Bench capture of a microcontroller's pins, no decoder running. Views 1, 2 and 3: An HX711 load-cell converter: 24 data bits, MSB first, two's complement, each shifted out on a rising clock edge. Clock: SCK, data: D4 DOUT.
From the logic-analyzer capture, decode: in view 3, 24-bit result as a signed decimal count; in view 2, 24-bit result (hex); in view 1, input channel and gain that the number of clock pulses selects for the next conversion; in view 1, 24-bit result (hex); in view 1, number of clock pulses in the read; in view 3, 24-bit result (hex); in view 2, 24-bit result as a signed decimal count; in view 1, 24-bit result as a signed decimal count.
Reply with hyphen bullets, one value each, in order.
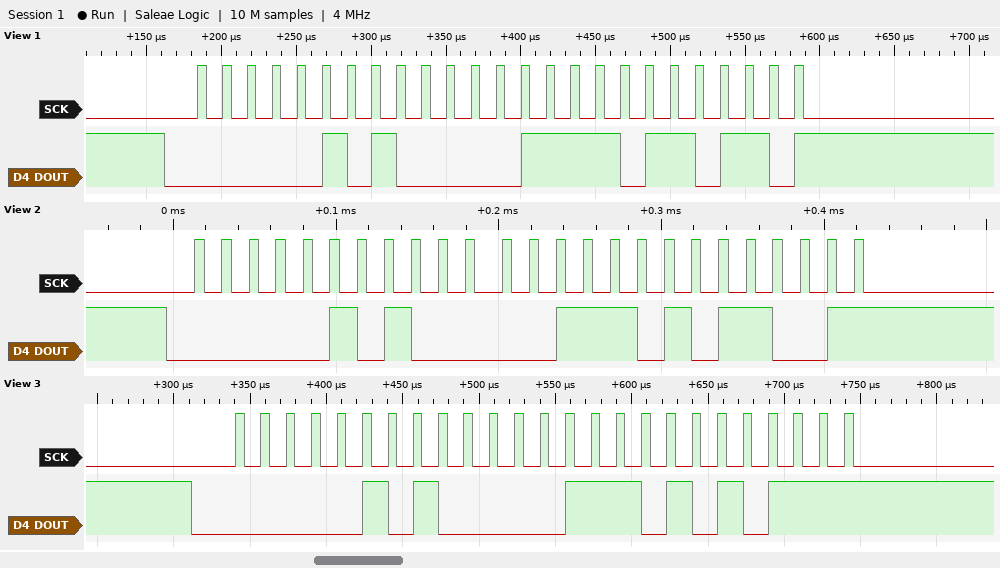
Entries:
- 329559
- 0x050759
- channel A, gain 128
- 0x0507B6
- 25
- 0x050757
- 329561
- 329654
